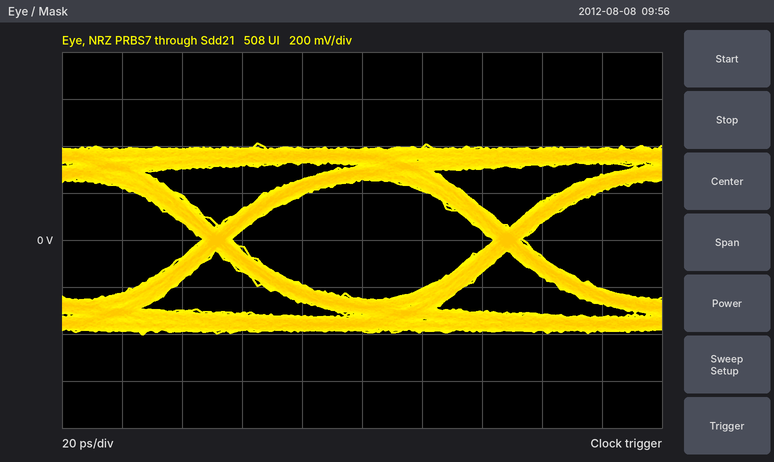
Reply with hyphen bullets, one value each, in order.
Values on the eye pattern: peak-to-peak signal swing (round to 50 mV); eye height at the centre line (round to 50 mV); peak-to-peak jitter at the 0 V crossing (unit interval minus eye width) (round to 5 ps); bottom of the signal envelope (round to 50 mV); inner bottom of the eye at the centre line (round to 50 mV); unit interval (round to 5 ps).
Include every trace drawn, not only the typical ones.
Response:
- 800 mV
- 500 mV
- 10 ps
- -400 mV
- -250 mV
- 95 ps
